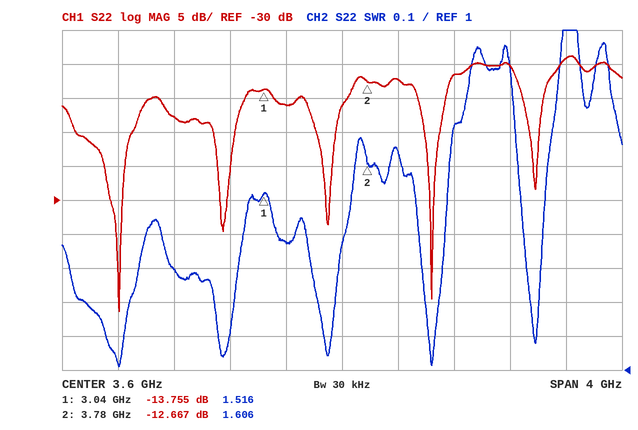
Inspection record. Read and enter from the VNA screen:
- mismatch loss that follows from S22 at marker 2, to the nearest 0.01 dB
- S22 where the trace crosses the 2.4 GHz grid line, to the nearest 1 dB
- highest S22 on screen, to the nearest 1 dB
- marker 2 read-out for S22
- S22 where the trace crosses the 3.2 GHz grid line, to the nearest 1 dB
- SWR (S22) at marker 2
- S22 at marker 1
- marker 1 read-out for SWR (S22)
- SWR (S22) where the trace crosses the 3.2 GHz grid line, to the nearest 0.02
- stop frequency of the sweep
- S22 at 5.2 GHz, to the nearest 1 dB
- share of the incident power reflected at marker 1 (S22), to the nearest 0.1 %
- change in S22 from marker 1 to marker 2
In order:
0.24 dB
-18 dB
-9 dB
-12.667 dB
-16 dB
1.606
-13.755 dB
1.516
1.38
5.6 GHz
-9 dB
4.2 %
1.088 dB
